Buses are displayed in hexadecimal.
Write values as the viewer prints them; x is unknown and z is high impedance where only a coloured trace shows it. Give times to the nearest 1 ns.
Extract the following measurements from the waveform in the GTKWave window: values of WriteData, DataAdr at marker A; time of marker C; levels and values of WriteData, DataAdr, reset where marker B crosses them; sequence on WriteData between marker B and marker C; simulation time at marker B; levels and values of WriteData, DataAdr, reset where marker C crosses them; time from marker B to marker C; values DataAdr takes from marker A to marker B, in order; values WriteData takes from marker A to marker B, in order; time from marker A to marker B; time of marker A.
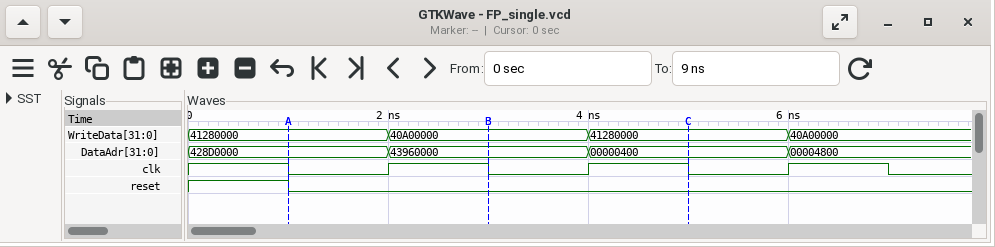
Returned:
WriteData=41280000, DataAdr=428D0000
5 ns
WriteData=40A00000, DataAdr=43960000, reset=0
40A00000, 41280000
3 ns
WriteData=41280000, DataAdr=00000400, reset=0
2 ns
428D0000, 43960000
41280000, 40A00000
2 ns
1 ns
